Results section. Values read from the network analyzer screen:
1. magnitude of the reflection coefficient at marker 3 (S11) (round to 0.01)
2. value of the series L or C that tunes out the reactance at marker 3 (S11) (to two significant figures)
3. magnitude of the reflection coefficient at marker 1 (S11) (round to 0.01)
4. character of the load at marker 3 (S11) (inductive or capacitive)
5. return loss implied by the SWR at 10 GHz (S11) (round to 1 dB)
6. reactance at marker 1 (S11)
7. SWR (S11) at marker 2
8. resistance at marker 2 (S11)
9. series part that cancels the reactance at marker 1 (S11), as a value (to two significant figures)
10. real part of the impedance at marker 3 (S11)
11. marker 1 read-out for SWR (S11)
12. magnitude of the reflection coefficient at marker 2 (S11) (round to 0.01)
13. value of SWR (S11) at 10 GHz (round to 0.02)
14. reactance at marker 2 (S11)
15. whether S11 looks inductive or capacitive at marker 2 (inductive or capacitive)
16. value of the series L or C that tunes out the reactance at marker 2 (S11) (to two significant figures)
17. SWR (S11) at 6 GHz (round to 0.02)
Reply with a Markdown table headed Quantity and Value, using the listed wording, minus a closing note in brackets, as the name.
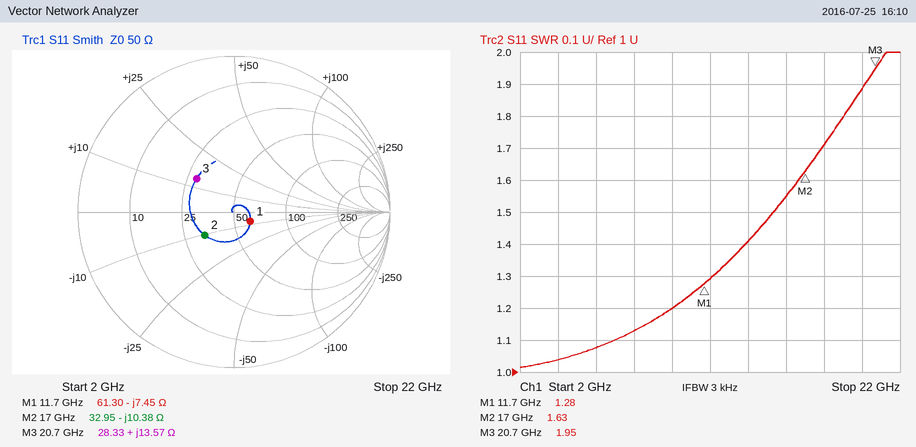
| Quantity | Value |
|---|---|
| magnitude of the reflection coefficient at marker 3 (S11) | 0.32 |
| value of the series L or C that tunes out the reactance at marker 3 (S11) | 570 fF |
| magnitude of the reflection coefficient at marker 1 (S11) | 0.12 |
| character of the load at marker 3 (S11) | inductive |
| return loss implied by the SWR at 10 GHz (S11) | 21 dB |
| reactance at marker 1 | -7.45 Ω |
| SWR (S11) at marker 2 | 1.63 |
| resistance at marker 2 | 32.95 Ω |
| series part that cancels the reactance at marker 1 (S11), as a value | 100 pH |
| real part of the impedance at marker 3 | 28.33 Ω |
| marker 1 read-out for SWR | 1.28 |
| magnitude of the reflection coefficient at marker 2 (S11) | 0.24 |
| value of SWR (S11) at 10 GHz | 1.20 |
| reactance at marker 2 | -10.38 Ω |
| whether S11 looks inductive or capacitive at marker 2 | capacitive |
| value of the series L or C that tunes out the reactance at marker 2 (S11) | 97 pH |
| SWR (S11) at 6 GHz | 1.08 |
